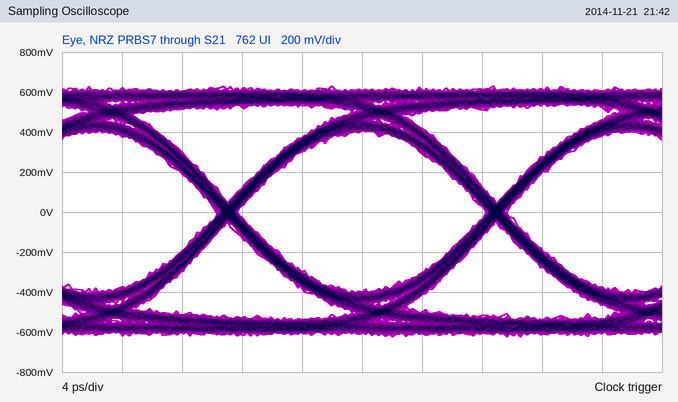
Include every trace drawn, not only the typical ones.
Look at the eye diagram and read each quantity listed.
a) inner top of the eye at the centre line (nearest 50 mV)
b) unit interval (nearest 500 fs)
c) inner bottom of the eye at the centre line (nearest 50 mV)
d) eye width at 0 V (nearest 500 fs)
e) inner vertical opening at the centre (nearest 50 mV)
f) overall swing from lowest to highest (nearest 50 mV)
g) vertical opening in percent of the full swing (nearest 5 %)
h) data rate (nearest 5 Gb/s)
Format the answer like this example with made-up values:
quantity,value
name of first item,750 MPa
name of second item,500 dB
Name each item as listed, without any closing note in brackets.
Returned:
quantity,value
inner top of the eye at the centre line,400 mV
unit interval,18.0 ps
inner bottom of the eye at the centre line,-400 mV
eye width at 0 V,16.5 ps
inner vertical opening at the centre,800 mV
overall swing from lowest to highest,1.25 V
vertical opening in percent of the full swing,65 %
data rate,55 Gb/s
